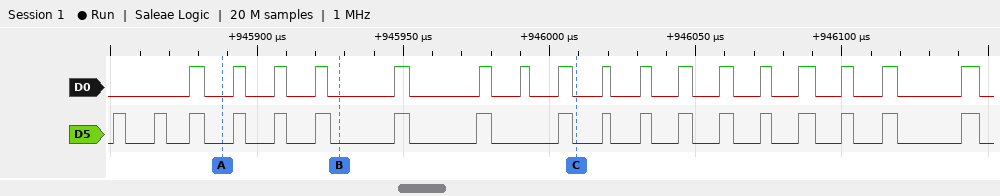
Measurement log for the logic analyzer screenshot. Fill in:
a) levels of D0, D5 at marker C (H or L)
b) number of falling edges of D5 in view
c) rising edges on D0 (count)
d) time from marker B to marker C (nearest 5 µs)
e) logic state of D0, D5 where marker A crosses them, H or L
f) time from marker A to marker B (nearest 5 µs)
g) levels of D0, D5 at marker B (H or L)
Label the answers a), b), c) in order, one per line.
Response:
a) D0=L, D5=L
b) 18
c) 17
d) 80 µs
e) D0=L, D5=L
f) 40 µs
g) D0=L, D5=L
